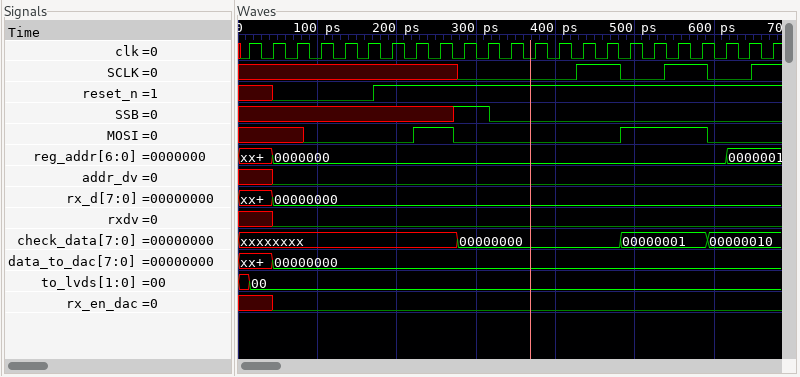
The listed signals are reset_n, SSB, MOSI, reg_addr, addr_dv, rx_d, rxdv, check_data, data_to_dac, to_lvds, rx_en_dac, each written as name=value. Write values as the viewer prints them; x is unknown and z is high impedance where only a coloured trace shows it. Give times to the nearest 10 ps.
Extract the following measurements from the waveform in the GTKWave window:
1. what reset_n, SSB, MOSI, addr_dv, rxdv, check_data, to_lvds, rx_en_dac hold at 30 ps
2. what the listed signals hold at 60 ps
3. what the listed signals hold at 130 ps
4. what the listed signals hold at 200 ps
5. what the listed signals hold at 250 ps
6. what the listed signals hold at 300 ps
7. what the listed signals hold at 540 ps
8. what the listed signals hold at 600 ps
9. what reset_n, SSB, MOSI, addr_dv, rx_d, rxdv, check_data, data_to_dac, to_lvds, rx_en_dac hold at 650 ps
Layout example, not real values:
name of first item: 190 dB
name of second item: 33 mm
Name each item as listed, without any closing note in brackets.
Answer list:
what reset_n, SSB, MOSI, addr_dv, rxdv, check_data, to_lvds, rx_en_dac hold at 30 ps: reset_n=x, SSB=x, MOSI=x, addr_dv=x, rxdv=x, check_data=xxxxxxxx, to_lvds=00, rx_en_dac=x
what the listed signals hold at 60 ps: reset_n=0, SSB=x, MOSI=x, reg_addr=0000000, addr_dv=0, rx_d=00000000, rxdv=0, check_data=xxxxxxxx, data_to_dac=00000000, to_lvds=00, rx_en_dac=0
what the listed signals hold at 130 ps: reset_n=0, SSB=x, MOSI=0, reg_addr=0000000, addr_dv=0, rx_d=00000000, rxdv=0, check_data=xxxxxxxx, data_to_dac=00000000, to_lvds=00, rx_en_dac=0
what the listed signals hold at 200 ps: reset_n=1, SSB=x, MOSI=0, reg_addr=0000000, addr_dv=0, rx_d=00000000, rxdv=0, check_data=xxxxxxxx, data_to_dac=00000000, to_lvds=00, rx_en_dac=0
what the listed signals hold at 250 ps: reset_n=1, SSB=x, MOSI=1, reg_addr=0000000, addr_dv=0, rx_d=00000000, rxdv=0, check_data=xxxxxxxx, data_to_dac=00000000, to_lvds=00, rx_en_dac=0
what the listed signals hold at 300 ps: reset_n=1, SSB=1, MOSI=0, reg_addr=0000000, addr_dv=0, rx_d=00000000, rxdv=0, check_data=00000000, data_to_dac=00000000, to_lvds=00, rx_en_dac=0
what the listed signals hold at 540 ps: reset_n=1, SSB=0, MOSI=1, reg_addr=0000000, addr_dv=0, rx_d=00000000, rxdv=0, check_data=00000001, data_to_dac=00000000, to_lvds=00, rx_en_dac=0
what the listed signals hold at 600 ps: reset_n=1, SSB=0, MOSI=0, reg_addr=0000000, addr_dv=0, rx_d=00000000, rxdv=0, check_data=00000010, data_to_dac=00000000, to_lvds=00, rx_en_dac=0
what reset_n, SSB, MOSI, addr_dv, rx_d, rxdv, check_data, data_to_dac, to_lvds, rx_en_dac hold at 650 ps: reset_n=1, SSB=0, MOSI=0, addr_dv=0, rx_d=00000000, rxdv=0, check_data=00000010, data_to_dac=00000000, to_lvds=00, rx_en_dac=0
